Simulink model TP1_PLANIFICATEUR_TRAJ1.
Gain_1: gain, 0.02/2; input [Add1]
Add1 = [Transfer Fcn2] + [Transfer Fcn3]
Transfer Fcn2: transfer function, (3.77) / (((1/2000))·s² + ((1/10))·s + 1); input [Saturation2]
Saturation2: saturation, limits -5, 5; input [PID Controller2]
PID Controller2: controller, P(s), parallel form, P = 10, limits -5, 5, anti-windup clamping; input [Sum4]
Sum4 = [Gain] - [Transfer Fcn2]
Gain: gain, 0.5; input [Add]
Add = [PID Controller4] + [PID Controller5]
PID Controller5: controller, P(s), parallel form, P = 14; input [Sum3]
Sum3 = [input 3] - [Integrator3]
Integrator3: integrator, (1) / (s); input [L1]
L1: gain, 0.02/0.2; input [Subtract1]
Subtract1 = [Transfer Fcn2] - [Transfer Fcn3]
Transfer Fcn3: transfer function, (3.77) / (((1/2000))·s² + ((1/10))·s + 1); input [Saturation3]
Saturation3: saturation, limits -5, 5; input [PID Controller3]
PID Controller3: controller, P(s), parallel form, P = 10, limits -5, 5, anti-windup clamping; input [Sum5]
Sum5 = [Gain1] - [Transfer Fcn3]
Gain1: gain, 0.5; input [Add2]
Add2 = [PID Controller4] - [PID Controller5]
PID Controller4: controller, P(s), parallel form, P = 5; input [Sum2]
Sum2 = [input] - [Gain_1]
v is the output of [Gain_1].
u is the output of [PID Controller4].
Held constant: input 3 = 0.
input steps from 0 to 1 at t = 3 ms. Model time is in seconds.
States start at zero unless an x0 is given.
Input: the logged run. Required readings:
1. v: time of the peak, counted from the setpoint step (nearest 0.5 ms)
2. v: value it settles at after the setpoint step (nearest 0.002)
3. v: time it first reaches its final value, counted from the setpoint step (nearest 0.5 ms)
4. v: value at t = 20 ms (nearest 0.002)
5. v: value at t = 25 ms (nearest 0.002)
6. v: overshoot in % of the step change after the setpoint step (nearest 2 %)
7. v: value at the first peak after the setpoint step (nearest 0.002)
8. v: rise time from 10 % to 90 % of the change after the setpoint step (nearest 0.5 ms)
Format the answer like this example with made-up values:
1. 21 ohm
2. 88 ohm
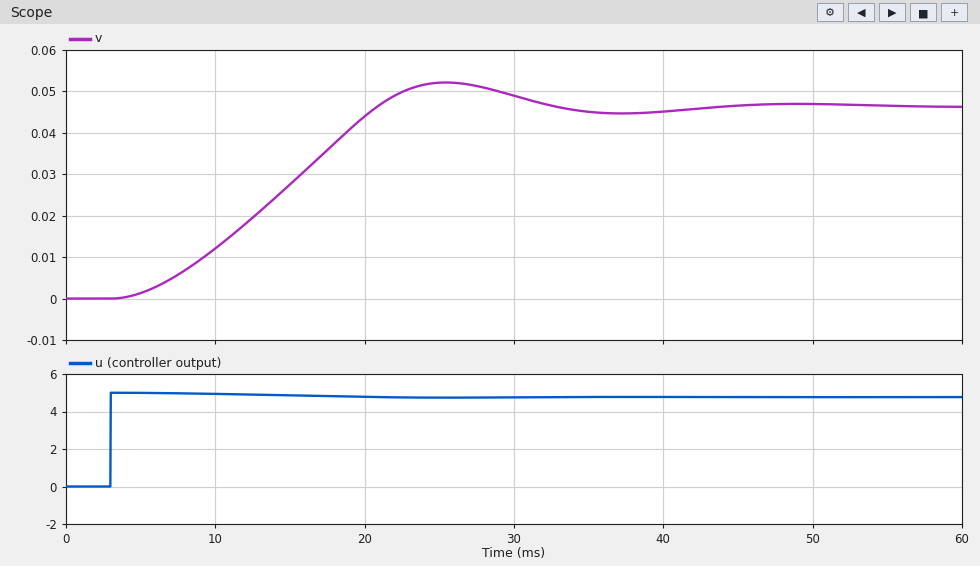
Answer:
1. 22.5 ms
2. 0.046
3. 18.0 ms
4. 0.044
5. 0.052
6. 12 %
7. 0.052
8. 12.5 ms
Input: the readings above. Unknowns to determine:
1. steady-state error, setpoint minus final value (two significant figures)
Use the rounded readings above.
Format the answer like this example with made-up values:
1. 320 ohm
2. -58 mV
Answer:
1. 0.95
